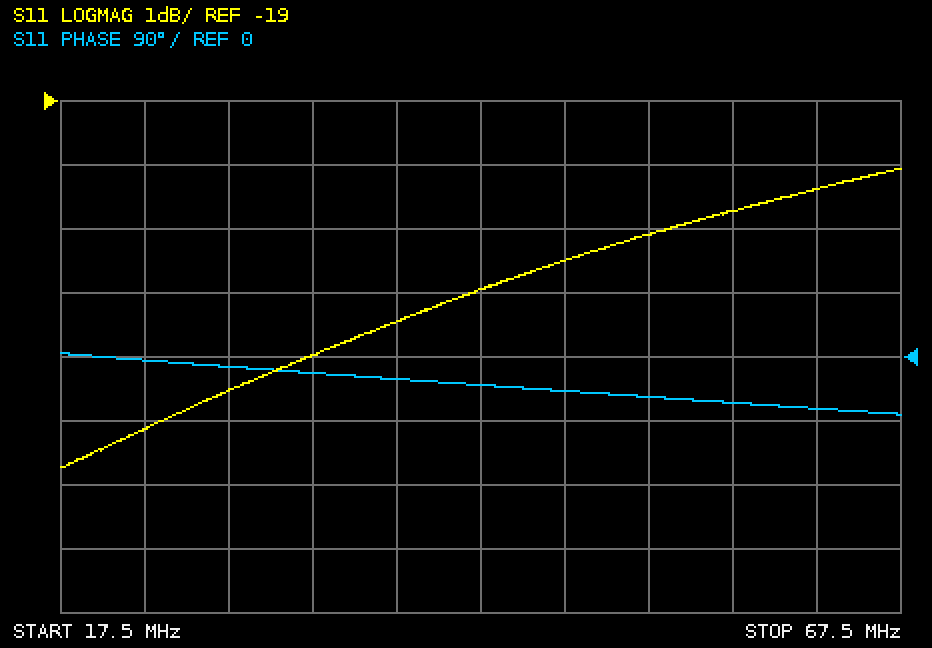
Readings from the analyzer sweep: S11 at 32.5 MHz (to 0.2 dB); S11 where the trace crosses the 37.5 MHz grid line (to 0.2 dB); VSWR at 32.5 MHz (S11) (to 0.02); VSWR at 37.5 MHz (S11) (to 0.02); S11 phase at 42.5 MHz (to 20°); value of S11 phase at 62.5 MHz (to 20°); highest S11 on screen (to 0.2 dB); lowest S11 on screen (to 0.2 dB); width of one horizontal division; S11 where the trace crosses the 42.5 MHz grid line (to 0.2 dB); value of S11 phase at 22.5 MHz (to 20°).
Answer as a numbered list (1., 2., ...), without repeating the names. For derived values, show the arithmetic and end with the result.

1. -23.0 dB
2. -22.4 dB
3. |Γ| = 10^(-23/20) = 0.0708; VSWR = (1 + 0.0708)/(1 − 0.0708) ≈ 1.15, so 1.16 to the nearest 0.02
4. |Γ| = 10^(-22.4/20) = 0.0759; VSWR = (1 + 0.0759)/(1 − 0.0759) ≈ 1.16
5. -40°
6. -80°
7. -20.0 dB
8. -24.8 dB
9. 5 MHz
10. -22.0 dB
11. 0°
